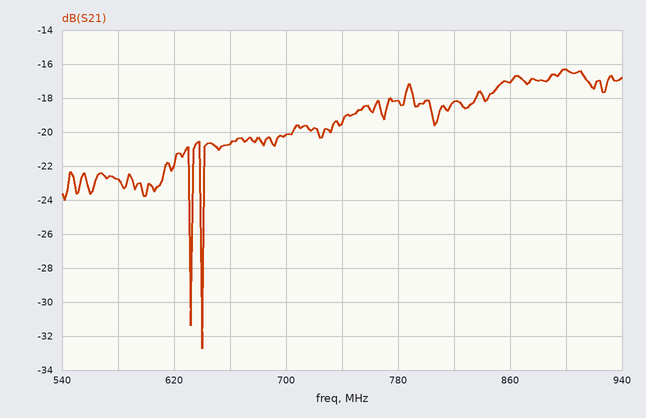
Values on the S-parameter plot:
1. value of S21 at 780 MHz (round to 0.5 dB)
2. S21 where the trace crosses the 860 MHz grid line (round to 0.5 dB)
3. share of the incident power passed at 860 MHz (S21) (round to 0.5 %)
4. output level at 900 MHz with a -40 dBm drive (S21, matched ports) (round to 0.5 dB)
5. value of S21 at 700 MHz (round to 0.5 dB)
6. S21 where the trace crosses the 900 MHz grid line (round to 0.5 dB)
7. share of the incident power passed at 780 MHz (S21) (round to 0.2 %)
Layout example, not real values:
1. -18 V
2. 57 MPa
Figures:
1. -18.0 dB
2. -17.0 dB
3. 2.0 %
4. -56.5 dBm
5. -20.0 dB
6. -16.5 dB
7. 1.6 %
